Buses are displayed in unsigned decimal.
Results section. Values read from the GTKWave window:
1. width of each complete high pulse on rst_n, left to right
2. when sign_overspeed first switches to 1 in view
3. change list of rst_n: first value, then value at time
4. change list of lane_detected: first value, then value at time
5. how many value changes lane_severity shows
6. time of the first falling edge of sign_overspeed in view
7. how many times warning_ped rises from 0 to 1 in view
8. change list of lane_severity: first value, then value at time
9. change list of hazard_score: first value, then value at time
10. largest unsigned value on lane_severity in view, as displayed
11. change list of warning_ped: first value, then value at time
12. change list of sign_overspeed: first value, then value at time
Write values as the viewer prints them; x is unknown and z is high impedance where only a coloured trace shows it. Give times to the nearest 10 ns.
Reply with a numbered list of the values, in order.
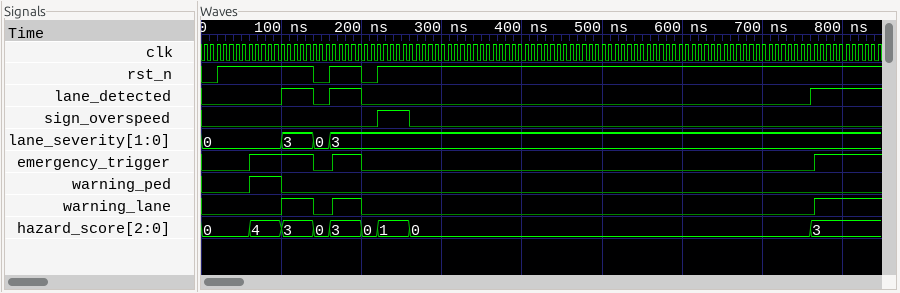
1. 120 ns, 40 ns
2. 220 ns
3. 0, 1 at 20 ns, 0 at 140 ns, 1 at 160 ns, 0 at 200 ns, 1 at 220 ns
4. 0, 1 at 100 ns, 0 at 140 ns, 1 at 160 ns, 0 at 200 ns, 1 at 760 ns
5. 3
6. 260 ns
7. 1
8. 0, 3 at 100 ns, 0 at 140 ns, 3 at 160 ns
9. 0, 4 at 60 ns, 3 at 100 ns, 0 at 140 ns, 3 at 160 ns, 0 at 200 ns, 1 at 220 ns, 0 at 260 ns, 3 at 760 ns
10. 3
11. 0, 1 at 60 ns, 0 at 100 ns
12. 0, 1 at 220 ns, 0 at 260 ns
